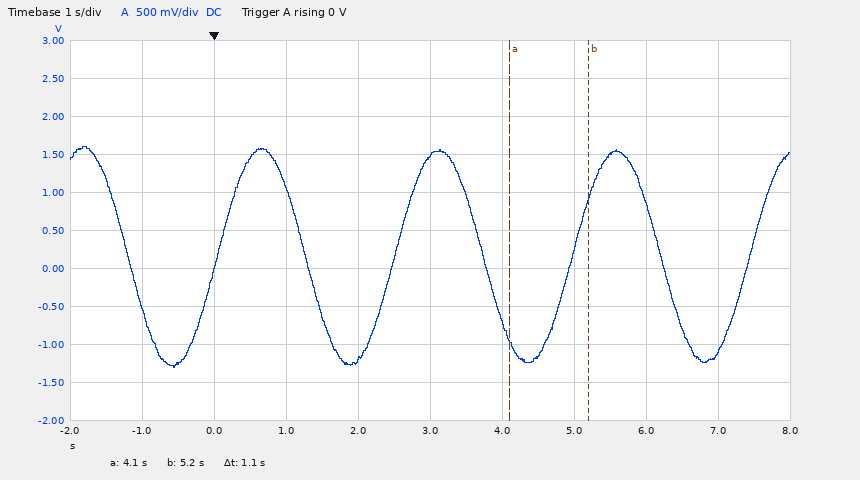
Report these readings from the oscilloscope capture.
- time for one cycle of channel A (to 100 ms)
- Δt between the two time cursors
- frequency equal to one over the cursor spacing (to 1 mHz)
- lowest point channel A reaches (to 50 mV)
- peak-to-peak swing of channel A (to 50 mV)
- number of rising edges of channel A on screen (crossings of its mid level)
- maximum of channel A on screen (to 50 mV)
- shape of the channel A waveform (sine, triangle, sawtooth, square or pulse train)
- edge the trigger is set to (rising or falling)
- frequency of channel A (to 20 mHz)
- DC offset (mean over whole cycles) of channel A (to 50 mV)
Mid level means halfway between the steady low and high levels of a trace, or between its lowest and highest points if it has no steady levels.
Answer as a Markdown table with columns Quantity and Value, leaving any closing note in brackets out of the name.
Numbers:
| Quantity | Value |
|---|---|
| time for one cycle of channel A | 2.5 s |
| Δt between the two time cursors | 1.1 s |
| frequency equal to one over the cursor spacing | 909 mHz |
| lowest point channel A reaches | -1.30 V |
| peak-to-peak swing of channel A | 2.90 V |
| number of rising edges of channel A on screen | 4 |
| maximum of channel A on screen | 1.60 V |
| shape of the channel A waveform | sine |
| edge the trigger is set to | rising |
| frequency of channel A | 400 mHz |
| DC offset (mean over whole cycles) of channel A | 150 mV |
